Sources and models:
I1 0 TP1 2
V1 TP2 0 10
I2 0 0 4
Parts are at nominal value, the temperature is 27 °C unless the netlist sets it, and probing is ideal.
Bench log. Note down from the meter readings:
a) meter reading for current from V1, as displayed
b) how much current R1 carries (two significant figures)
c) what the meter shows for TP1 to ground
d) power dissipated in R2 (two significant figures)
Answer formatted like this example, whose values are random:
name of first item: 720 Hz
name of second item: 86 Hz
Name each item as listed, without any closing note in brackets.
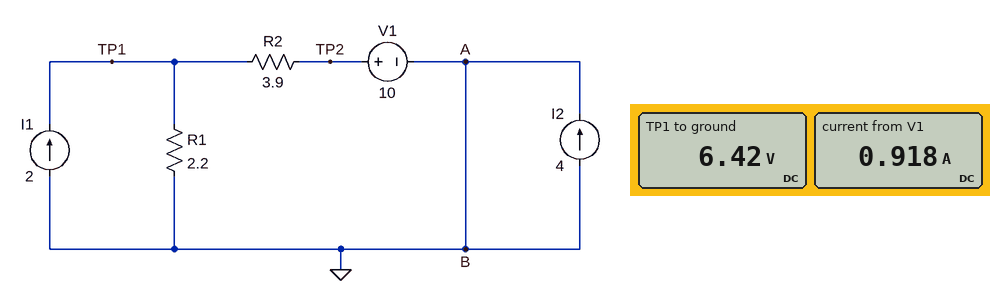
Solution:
meter reading for current from V1, as displayed: 0.918 A
how much current R1 carries: 2.9 A
what the meter shows for TP1 to ground: 6.42 V
power dissipated in R2: 3.3 W
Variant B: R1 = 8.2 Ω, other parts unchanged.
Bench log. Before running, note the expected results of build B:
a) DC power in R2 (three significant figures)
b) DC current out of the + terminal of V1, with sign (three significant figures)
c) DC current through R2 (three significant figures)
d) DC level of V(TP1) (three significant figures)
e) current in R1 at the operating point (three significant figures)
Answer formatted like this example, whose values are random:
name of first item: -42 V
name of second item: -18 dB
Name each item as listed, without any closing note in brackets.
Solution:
DC power in R2: 1.09 W
DC current out of the + terminal of V1, with sign: -529 mA
DC current through R2: 529 mA
DC level of V(TP1): 12.1 V
current in R1 at the operating point: 1.47 A
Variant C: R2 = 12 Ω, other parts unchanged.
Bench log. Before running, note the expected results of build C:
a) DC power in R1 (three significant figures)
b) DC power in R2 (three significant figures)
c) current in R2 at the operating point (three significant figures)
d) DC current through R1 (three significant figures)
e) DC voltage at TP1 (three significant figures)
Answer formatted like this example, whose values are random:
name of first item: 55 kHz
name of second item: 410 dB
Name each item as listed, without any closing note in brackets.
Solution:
DC power in R1: 12.6 W
DC power in R2: 1.87 W
current in R2 at the operating point: 394 mA
DC current through R1: 2.39 A
DC voltage at TP1: 5.27 V
